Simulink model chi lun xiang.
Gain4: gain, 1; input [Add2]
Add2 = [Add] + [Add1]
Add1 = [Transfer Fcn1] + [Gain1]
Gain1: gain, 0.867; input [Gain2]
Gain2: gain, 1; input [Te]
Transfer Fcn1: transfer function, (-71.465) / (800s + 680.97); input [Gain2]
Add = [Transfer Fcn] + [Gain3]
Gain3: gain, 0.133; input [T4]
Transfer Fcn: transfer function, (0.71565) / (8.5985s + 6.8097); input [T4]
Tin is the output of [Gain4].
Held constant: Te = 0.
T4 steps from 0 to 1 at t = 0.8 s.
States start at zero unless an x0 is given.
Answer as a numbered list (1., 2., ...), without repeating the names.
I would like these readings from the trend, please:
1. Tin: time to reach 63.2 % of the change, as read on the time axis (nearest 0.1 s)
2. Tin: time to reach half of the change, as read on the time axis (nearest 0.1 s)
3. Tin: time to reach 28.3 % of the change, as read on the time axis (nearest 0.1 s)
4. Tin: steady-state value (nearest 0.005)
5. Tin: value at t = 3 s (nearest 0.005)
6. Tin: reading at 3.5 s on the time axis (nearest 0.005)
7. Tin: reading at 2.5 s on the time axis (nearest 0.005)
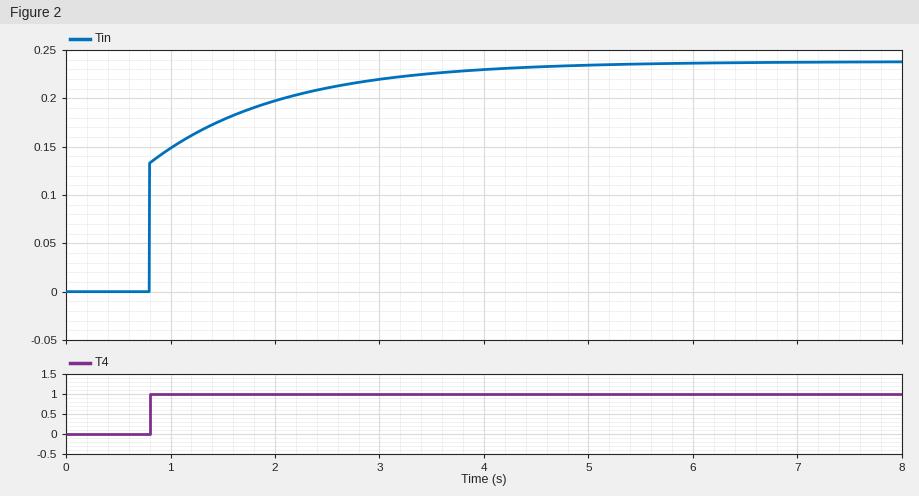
1. 1.0 s
2. 0.8 s
3. 0.8 s
4. 0.240
5. 0.220
6. 0.225
7. 0.210
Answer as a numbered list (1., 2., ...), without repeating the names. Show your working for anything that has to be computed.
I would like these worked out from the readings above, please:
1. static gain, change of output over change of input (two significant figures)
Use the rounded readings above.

1. (0.24 - 0) / (1 - 0) = 0.24
